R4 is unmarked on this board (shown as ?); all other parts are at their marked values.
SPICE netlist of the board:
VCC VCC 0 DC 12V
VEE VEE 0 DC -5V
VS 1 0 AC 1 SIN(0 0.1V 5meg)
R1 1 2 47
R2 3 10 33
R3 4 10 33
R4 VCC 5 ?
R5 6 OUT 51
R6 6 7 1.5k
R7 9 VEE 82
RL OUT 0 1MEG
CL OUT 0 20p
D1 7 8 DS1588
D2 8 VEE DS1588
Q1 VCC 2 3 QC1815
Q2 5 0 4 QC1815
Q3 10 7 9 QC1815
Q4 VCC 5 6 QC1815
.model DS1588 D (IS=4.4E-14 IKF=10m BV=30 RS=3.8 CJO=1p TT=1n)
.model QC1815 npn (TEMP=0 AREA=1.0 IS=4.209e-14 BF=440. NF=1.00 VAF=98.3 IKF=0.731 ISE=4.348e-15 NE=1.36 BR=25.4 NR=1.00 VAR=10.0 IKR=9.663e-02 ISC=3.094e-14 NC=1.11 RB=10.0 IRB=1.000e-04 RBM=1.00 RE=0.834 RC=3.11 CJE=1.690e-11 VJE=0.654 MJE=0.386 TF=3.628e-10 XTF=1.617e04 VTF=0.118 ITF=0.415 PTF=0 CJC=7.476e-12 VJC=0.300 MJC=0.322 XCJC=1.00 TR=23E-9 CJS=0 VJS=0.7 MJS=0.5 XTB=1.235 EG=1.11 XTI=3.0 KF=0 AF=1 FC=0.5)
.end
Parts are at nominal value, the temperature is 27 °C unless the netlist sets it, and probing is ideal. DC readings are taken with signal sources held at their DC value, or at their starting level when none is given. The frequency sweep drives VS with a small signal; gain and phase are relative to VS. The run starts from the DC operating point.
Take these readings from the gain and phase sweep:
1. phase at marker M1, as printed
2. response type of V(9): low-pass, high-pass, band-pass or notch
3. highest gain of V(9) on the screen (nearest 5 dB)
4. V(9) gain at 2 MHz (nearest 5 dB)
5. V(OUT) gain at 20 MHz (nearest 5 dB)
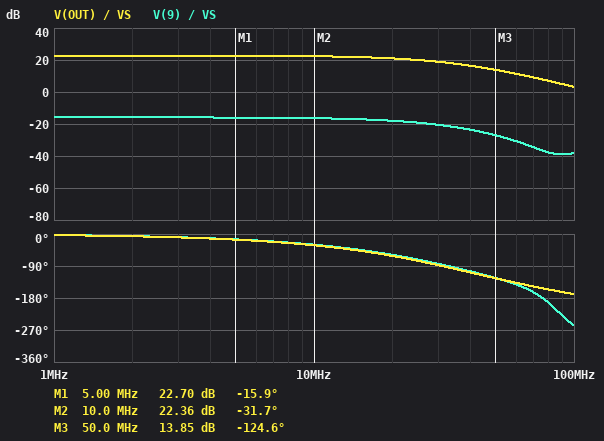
-15.9 deg
low-pass
-15 dB
-15 dB
20 dB
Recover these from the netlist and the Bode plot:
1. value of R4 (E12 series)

1.2 kΩ
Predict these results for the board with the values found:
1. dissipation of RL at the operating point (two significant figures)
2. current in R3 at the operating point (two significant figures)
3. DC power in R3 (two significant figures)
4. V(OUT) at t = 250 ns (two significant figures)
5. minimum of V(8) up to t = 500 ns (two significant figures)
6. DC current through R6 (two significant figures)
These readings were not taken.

39 µW
4.2 mA
580 µW
7.5 V
-4.3 V
6.5 mA
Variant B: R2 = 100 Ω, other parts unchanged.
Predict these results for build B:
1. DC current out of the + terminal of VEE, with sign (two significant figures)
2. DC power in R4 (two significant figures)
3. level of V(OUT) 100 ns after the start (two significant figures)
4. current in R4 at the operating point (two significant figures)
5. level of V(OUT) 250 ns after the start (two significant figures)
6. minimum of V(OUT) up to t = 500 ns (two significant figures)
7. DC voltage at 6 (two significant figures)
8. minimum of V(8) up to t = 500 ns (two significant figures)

-13 mA
42 mW
4.4 V
5.9 mA
4.9 V
3.5 V
4.2 V
-4.3 V
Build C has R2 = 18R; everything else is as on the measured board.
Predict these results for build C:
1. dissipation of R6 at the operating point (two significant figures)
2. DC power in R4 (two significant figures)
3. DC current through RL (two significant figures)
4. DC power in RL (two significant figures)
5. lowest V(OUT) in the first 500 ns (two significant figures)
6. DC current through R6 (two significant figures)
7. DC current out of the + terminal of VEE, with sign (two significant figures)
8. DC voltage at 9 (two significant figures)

79 mW
13 mW
7.3 µA
54 µW
5.6 V
7.3 mA
-16 mA
-4.3 V
